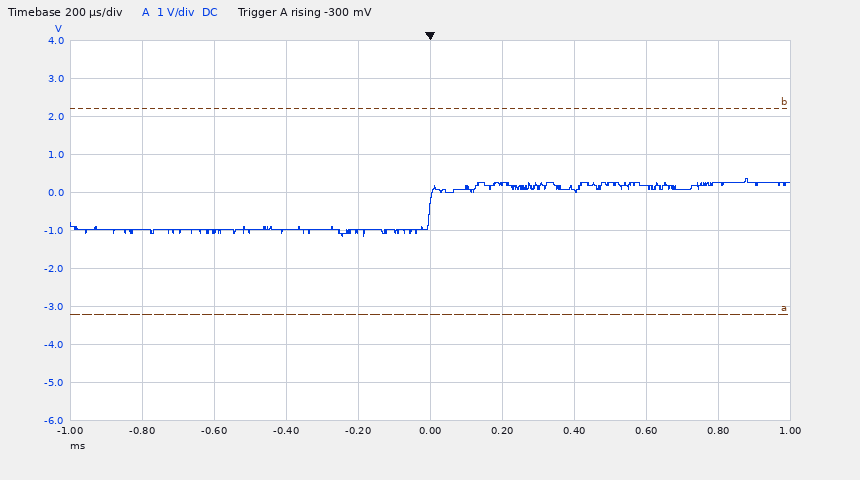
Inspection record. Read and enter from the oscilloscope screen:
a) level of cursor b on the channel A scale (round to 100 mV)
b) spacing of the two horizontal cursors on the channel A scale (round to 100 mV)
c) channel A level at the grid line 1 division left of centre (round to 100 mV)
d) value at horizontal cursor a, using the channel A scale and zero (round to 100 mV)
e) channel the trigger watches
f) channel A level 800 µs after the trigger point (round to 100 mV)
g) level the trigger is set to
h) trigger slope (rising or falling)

2.2 V
5.4 V
-1.0 V
-3.2 V
channel A
300 mV
-300 mV
rising
